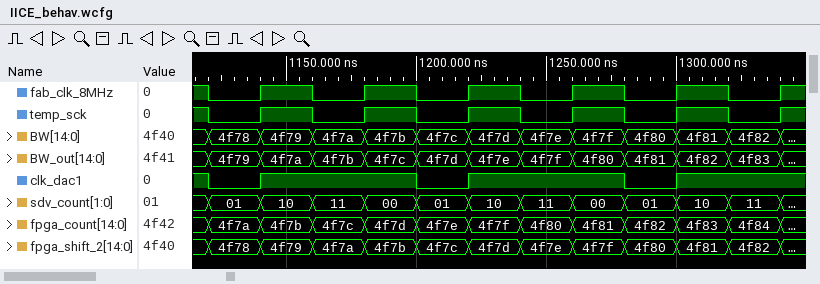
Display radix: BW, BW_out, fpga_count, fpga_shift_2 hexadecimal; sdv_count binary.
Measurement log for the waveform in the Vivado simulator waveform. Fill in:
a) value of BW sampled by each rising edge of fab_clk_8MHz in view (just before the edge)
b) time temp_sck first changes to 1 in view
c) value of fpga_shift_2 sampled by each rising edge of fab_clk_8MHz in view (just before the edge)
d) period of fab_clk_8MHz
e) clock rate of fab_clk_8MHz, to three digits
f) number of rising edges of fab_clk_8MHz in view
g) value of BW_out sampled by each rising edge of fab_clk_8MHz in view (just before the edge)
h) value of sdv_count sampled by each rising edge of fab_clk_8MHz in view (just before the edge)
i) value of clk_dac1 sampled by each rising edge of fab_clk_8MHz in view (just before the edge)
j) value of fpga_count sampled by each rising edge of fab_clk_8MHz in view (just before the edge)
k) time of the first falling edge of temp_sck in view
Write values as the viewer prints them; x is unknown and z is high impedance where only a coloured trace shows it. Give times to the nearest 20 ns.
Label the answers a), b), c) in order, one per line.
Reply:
a) 4f78, 4f7a, 4f7c, 4f7e, 4f80, 4f82
b) 1140 ns
c) 4f78, 4f7a, 4f7c, 4f7e, 4f80, 4f82
d) 40 ns
e) 25.0 MHz
f) 6
g) 4f79, 4f7b, 4f7d, 4f7f, 4f81, 4f83
h) 01, 11, 01, 11, 01, 11
i) 0 1 0 1 0 1
j) 4f7a, 4f7c, 4f7e, 4f80, 4f82, 4f84
k) 1120 ns
